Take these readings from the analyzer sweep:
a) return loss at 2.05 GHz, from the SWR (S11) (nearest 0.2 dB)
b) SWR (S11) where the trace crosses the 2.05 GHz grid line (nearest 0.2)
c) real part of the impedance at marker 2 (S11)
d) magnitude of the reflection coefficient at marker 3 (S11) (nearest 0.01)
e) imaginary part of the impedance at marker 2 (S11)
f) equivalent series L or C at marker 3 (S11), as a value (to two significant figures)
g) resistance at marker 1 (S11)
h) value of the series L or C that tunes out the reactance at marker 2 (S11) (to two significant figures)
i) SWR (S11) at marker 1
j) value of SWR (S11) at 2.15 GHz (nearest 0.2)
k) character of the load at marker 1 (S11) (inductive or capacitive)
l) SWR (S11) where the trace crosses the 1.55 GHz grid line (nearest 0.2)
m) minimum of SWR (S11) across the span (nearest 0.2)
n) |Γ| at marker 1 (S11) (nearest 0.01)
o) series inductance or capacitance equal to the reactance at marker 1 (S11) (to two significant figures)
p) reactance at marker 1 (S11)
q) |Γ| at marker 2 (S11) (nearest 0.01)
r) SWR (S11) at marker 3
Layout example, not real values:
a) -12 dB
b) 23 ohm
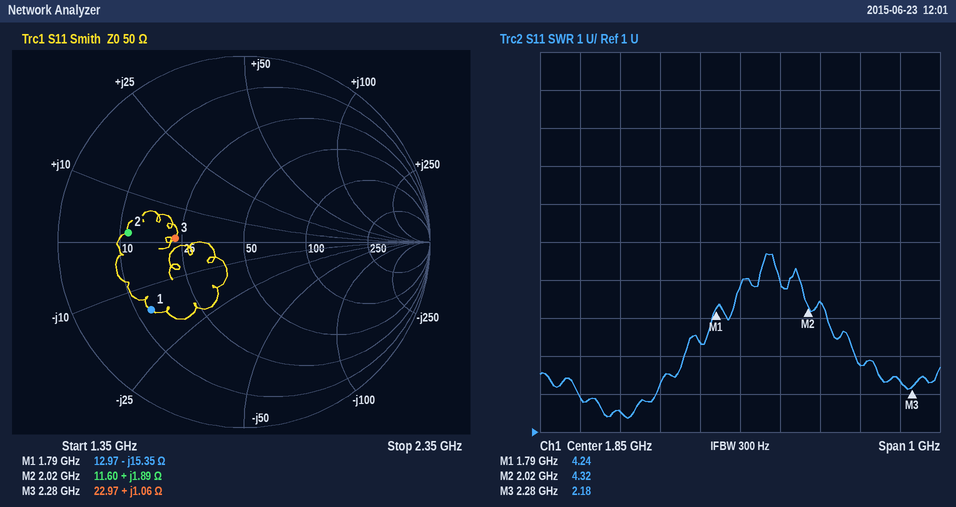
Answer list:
a) 4.0 dB
b) 4.4
c) 11.60 Ω
d) 0.37
e) +1.89 Ω
f) 74 pH
g) 12.97 Ω
h) 42 pF
i) 4.24
j) 2.8
k) capacitive
l) 1.6
m) 1.4
n) 0.62
o) 5.8 pF
p) -15.35 Ω
q) 0.62
r) 2.18
